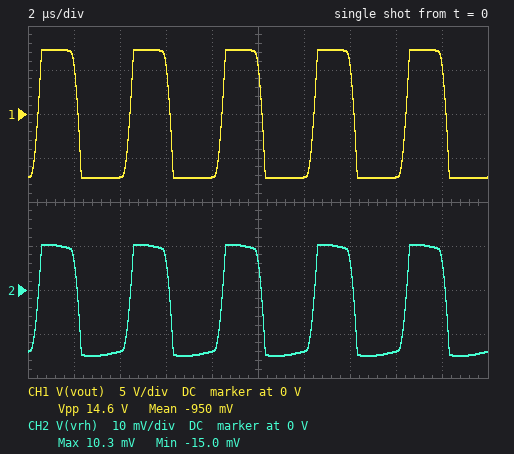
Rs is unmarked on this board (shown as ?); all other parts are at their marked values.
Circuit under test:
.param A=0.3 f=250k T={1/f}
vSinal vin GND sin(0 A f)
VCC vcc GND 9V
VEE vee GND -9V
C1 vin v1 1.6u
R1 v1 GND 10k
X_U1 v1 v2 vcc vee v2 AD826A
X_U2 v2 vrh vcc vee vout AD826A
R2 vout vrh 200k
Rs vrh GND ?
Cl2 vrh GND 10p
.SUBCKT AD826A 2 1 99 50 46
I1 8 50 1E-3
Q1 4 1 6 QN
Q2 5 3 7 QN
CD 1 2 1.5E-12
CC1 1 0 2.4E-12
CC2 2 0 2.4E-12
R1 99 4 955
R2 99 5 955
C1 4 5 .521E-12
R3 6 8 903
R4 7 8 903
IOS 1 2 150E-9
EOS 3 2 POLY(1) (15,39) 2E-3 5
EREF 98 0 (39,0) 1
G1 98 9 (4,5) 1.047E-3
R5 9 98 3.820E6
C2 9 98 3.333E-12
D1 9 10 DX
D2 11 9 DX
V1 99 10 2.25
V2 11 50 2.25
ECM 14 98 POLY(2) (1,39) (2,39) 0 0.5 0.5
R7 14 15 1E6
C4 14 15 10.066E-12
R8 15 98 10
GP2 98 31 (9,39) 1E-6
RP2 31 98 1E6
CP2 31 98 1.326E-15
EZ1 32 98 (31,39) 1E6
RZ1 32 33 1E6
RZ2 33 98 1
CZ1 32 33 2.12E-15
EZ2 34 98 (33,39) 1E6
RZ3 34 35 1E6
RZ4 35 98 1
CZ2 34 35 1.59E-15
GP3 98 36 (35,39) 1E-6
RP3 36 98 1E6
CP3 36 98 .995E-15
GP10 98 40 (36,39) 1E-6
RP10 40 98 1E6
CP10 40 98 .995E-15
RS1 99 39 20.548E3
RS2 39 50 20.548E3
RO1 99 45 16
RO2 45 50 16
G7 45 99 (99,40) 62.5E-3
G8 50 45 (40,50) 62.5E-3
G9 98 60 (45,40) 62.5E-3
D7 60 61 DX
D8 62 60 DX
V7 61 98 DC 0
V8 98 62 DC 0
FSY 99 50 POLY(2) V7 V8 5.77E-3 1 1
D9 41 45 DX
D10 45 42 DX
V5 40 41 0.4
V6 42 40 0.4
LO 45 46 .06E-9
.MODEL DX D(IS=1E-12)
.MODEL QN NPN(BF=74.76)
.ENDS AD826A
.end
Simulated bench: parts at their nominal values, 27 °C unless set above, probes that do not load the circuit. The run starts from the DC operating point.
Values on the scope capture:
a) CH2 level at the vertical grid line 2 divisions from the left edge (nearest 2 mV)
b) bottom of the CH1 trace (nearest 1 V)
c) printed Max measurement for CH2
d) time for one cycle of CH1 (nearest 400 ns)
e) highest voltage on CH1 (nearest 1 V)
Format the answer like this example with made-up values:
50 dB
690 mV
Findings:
-14 mV
-7 V
10.3 mV
4.0 µs
7 V
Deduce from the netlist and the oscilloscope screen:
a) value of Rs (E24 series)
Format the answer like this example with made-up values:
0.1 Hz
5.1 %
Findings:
330 Ω
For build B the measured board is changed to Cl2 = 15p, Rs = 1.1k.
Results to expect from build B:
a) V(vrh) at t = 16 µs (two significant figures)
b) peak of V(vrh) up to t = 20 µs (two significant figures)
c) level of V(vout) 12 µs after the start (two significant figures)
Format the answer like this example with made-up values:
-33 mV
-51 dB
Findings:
-46 mV
34 mV
-7.2 V
